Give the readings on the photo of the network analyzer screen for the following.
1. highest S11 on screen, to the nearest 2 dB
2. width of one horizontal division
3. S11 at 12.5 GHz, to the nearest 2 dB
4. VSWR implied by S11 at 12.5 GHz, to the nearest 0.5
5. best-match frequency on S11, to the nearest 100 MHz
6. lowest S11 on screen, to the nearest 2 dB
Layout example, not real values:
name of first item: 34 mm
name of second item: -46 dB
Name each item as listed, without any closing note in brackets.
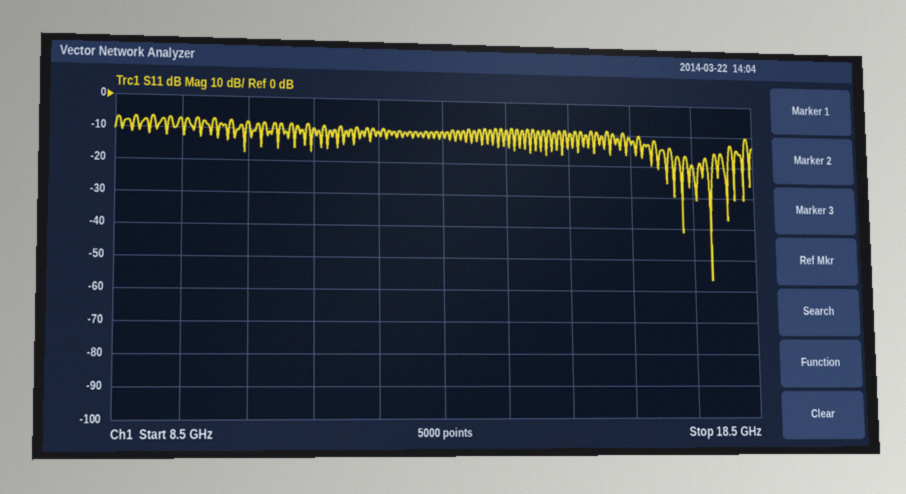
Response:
highest S11 on screen, to the nearest 2 dB: -6 dB
width of one horizontal division: 1 GHz
S11 at 12.5 GHz, to the nearest 2 dB: -10 dB
VSWR implied by S11 at 12.5 GHz, to the nearest 0.5: 2.0
best-match frequency on S11, to the nearest 100 MHz: 17.8 GHz
lowest S11 on screen, to the nearest 2 dB: -56 dB
